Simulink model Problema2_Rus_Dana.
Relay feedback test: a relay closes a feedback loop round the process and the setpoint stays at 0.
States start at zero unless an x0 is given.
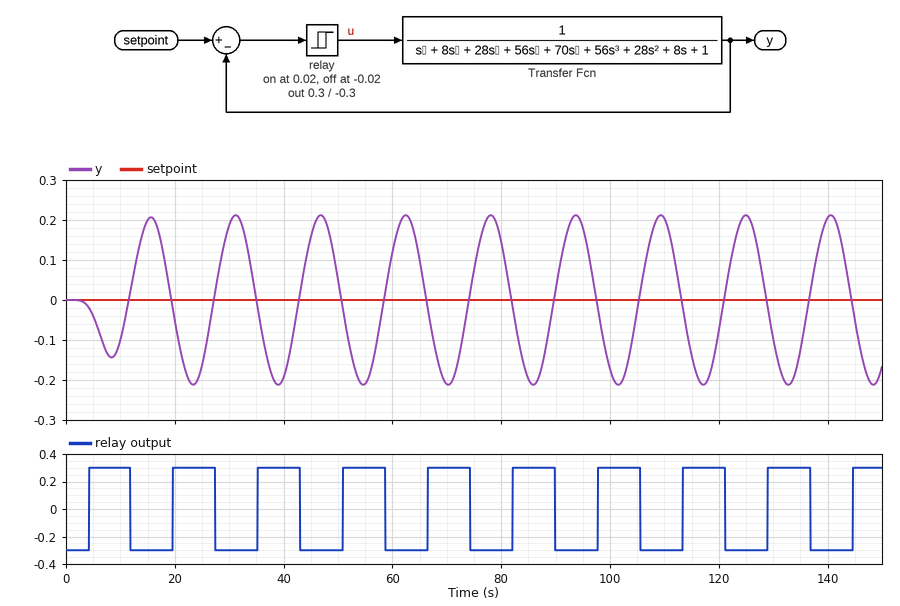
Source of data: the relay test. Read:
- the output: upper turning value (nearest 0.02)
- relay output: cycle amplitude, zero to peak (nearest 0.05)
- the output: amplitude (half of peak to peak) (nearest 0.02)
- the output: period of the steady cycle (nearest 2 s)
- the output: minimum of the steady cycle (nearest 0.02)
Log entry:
0.22
0.30
0.22
16 s
-0.22
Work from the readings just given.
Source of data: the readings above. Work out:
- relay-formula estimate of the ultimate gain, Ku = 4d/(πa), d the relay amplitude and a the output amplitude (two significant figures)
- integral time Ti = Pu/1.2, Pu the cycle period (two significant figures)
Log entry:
1.7
13 s
